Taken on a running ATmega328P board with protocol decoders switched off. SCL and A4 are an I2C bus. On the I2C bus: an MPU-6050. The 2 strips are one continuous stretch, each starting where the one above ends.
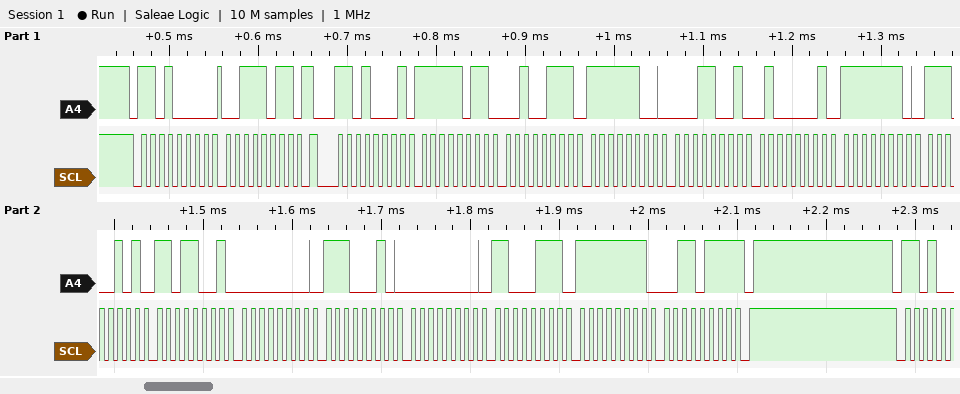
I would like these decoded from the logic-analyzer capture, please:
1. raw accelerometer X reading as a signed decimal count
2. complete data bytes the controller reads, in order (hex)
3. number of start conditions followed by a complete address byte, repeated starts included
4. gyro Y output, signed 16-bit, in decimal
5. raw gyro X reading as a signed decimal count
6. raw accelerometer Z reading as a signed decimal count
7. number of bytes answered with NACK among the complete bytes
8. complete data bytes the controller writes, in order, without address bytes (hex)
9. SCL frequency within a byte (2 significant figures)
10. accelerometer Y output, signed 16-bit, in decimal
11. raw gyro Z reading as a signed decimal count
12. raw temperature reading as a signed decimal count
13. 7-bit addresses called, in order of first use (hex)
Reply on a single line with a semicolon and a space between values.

-1241; FB 27 FC 19 41 FE E5 D9 00 E2 00 C7 FF 37; 2; 199; 226; 16894; 1; 3B; 100 kHz; -999; -201; -6695; 0x68
